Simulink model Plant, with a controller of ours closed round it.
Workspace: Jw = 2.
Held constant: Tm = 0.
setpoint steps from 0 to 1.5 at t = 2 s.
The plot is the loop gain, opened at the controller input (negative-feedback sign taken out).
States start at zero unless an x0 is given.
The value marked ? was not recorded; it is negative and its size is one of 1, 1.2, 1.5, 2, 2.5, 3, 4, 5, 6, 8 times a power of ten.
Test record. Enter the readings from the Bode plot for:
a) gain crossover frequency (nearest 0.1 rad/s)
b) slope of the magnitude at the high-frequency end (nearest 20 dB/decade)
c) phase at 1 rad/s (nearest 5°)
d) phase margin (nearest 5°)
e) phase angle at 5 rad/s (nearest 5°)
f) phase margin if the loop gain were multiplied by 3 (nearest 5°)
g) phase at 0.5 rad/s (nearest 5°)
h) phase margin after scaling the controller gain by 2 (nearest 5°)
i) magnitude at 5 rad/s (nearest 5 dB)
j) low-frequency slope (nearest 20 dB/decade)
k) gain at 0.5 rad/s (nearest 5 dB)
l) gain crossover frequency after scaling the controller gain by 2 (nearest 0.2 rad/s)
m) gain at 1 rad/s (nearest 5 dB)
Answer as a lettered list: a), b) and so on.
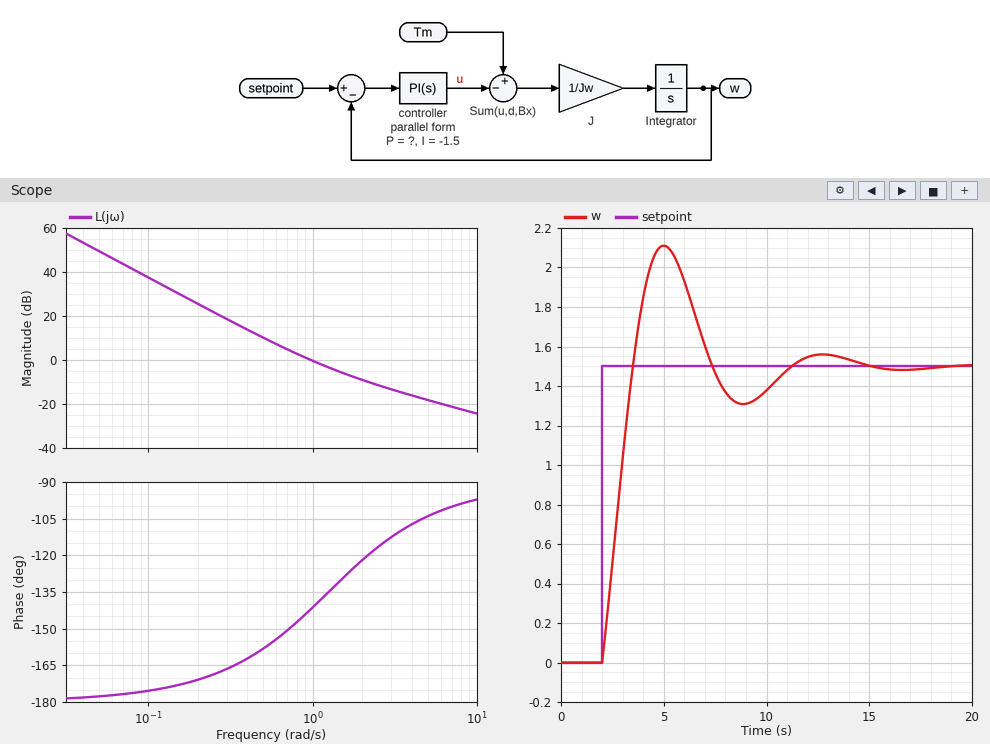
a) 1.0 rad/s
b) -20 dB/decade
c) -140°
d) 40°
e) -105°
f) 60°
g) -160°
h) 50°
i) -20 dB
j) -40 dB/decade
k) 10 dB
l) 1.6 rad/s
m) 0 dB
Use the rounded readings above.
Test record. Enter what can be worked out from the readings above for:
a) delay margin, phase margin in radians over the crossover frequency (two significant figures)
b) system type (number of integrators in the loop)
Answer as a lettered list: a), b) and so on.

a) 0.70 s
b) 2
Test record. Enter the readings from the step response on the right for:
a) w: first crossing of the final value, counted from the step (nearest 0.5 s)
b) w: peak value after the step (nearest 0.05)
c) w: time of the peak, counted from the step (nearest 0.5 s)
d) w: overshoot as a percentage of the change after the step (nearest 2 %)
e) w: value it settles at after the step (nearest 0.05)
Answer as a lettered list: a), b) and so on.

a) 1.5 s
b) 2.10
c) 3.0 s
d) 40 %
e) 1.50
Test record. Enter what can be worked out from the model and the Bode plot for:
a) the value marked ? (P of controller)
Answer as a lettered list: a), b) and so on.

a) -1.2
